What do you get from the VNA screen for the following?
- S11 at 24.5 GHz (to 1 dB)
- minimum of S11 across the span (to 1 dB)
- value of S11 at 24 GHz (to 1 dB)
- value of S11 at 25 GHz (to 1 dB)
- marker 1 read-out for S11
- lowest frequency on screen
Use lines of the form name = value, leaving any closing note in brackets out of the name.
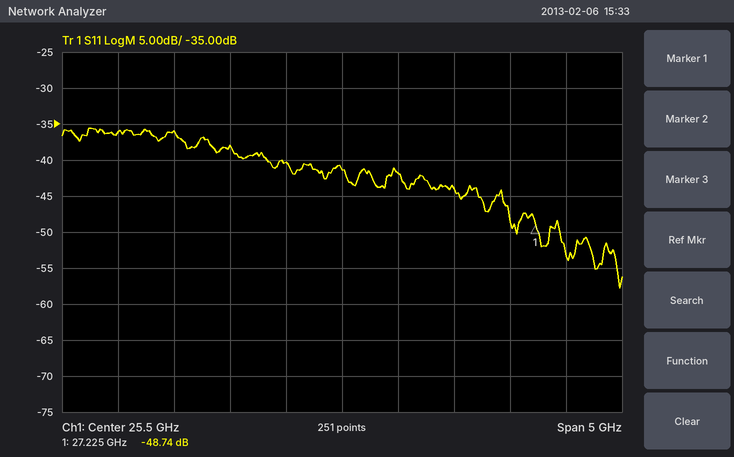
S11 at 24.5 GHz = -38 dB
minimum of S11 across the span = -58 dB
value of S11 at 24 GHz = -36 dB
value of S11 at 25 GHz = -40 dB
marker 1 read-out for S11 = -48.74 dB
lowest frequency on screen = 23 GHz
